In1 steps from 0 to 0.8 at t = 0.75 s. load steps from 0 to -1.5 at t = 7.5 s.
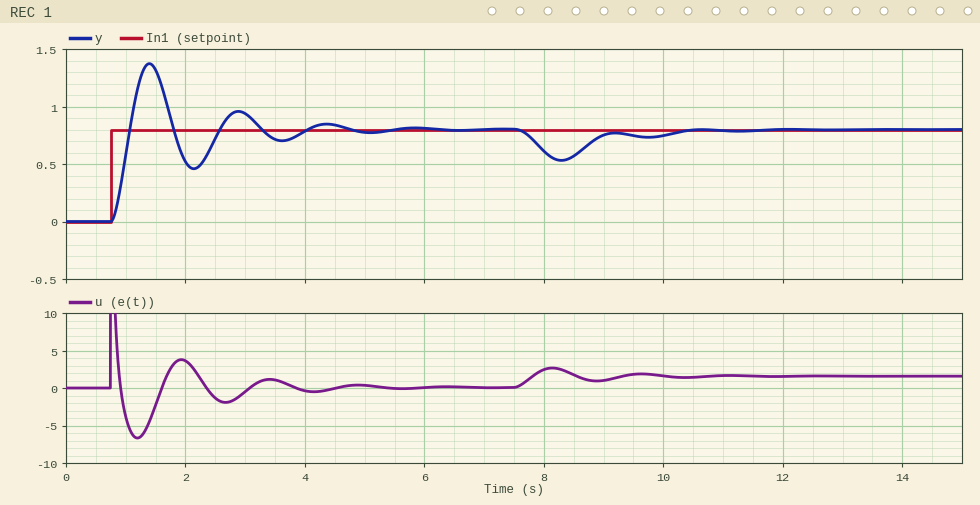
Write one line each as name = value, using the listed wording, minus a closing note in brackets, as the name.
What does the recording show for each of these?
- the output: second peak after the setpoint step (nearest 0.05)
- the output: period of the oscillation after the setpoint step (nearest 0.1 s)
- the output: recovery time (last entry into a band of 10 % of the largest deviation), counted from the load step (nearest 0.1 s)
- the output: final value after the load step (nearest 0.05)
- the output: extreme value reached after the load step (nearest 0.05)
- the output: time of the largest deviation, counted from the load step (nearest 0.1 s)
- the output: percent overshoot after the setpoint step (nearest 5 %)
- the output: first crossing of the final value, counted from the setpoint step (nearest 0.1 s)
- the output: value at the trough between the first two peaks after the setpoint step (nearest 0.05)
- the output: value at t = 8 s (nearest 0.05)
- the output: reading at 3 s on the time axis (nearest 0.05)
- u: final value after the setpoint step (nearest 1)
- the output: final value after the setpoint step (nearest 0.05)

the output: second peak after the setpoint step = 0.95
the output: period of the oscillation after the setpoint step = 1.5 s
the output: recovery time (last entry into a band of 10 % of the largest deviation), counted from the load step = 2.7 s
the output: final value after the load step = 0.80
the output: extreme value reached after the load step = 0.55
the output: time of the largest deviation, counted from the load step = 0.8 s
the output: percent overshoot after the setpoint step = 70 %
the output: first crossing of the final value, counted from the setpoint step = 0.3 s
the output: value at the trough between the first two peaks after the setpoint step = 0.45
the output: value at t = 8 s = 0.60
the output: reading at 3 s on the time axis = 0.95
u: final value after the setpoint step = 0
the output: final value after the setpoint step = 0.80
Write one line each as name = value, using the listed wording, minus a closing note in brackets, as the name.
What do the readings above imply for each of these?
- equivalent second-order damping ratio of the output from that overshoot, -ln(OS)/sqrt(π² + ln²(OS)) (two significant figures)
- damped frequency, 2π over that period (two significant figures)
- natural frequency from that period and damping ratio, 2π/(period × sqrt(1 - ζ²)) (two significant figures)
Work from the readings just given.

equivalent second-order damping ratio of the output from that overshoot, -ln(OS)/sqrt(π² + ln²(OS)) = 0.11
damped frequency, 2π over that period = 4.2 rad/s
natural frequency from that period and damping ratio, 2π/(period × sqrt(1 - ζ²)) = 4.2 rad/s
